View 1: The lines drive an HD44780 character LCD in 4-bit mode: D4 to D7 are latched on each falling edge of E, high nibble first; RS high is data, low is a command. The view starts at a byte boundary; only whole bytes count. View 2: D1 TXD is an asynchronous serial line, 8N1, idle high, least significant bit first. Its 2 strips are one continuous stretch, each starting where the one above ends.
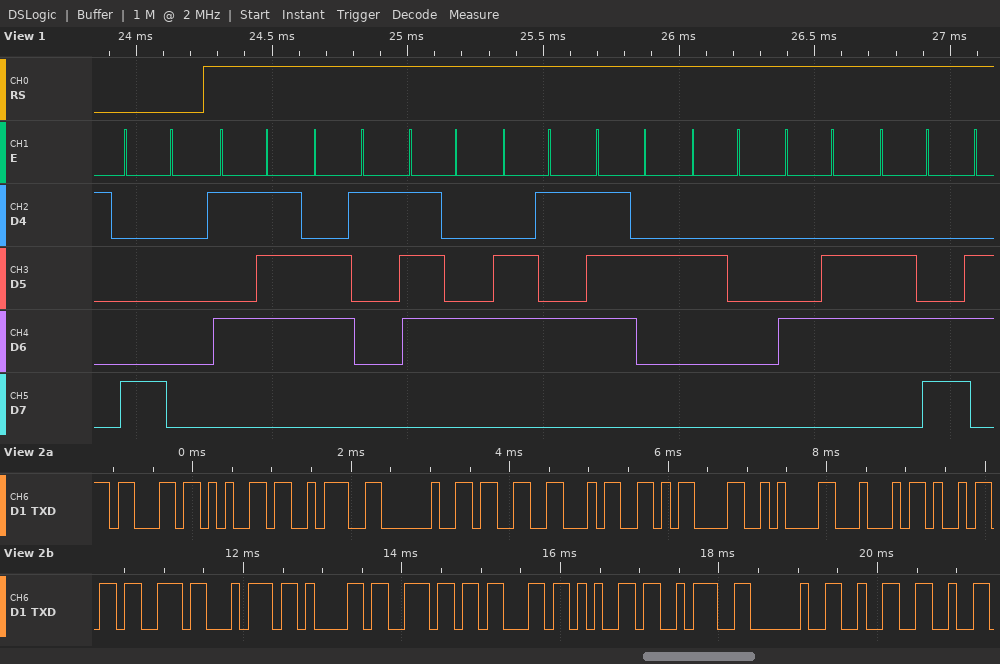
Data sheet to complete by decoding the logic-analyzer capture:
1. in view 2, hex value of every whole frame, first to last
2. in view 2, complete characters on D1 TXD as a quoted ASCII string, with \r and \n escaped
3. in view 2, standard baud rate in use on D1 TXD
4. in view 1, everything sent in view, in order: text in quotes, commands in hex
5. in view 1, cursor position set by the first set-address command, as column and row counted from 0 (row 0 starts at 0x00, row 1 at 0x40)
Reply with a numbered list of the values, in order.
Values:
1. 63 65 3A 20 33 34 0D 0A 44 69 73 74 61 6E 63 65 3A 20 32
2. "ce: 34\r\nDistance: 2"
3. 9600 baud
4. 0x80 "Water Fl"
5. column 0, row 0
